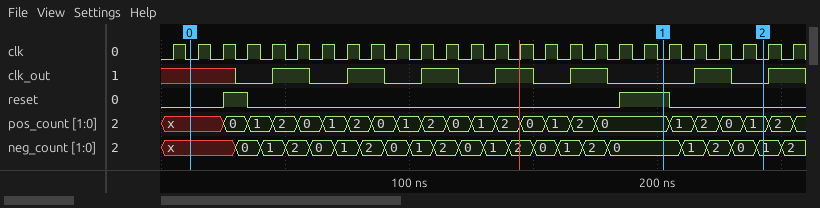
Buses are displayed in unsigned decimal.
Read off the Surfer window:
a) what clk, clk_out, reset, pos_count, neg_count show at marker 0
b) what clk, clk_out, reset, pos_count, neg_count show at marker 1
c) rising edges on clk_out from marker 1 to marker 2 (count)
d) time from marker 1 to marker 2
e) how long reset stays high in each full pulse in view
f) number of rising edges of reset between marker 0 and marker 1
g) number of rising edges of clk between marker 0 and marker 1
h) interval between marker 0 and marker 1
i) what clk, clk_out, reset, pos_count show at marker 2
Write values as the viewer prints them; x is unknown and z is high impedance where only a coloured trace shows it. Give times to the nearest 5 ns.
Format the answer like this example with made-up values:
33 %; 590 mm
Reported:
clk=0, clk_out=x, reset=0, pos_count=x, neg_count=x; clk=0, clk_out=0, reset=1, pos_count=0, neg_count=0; 1; 40 ns; 10 ns, 20 ns; 2; 19; 190 ns; clk=0, clk_out=0, reset=0, pos_count=1
